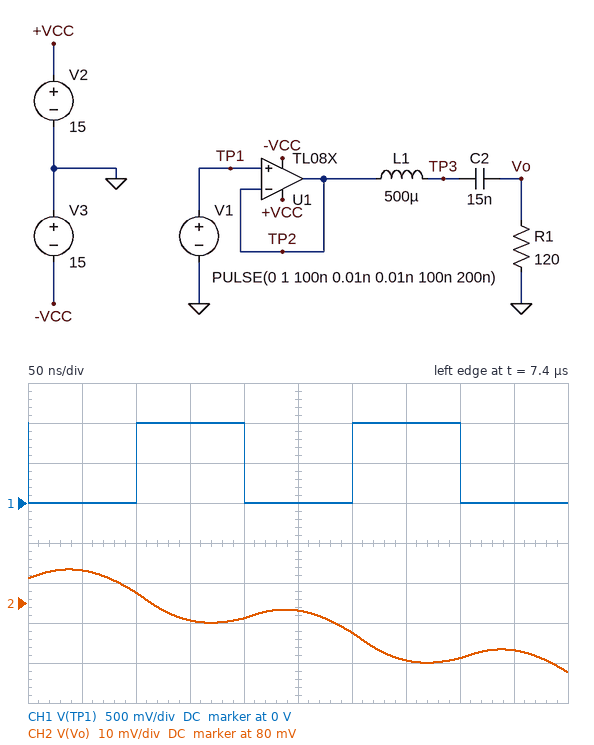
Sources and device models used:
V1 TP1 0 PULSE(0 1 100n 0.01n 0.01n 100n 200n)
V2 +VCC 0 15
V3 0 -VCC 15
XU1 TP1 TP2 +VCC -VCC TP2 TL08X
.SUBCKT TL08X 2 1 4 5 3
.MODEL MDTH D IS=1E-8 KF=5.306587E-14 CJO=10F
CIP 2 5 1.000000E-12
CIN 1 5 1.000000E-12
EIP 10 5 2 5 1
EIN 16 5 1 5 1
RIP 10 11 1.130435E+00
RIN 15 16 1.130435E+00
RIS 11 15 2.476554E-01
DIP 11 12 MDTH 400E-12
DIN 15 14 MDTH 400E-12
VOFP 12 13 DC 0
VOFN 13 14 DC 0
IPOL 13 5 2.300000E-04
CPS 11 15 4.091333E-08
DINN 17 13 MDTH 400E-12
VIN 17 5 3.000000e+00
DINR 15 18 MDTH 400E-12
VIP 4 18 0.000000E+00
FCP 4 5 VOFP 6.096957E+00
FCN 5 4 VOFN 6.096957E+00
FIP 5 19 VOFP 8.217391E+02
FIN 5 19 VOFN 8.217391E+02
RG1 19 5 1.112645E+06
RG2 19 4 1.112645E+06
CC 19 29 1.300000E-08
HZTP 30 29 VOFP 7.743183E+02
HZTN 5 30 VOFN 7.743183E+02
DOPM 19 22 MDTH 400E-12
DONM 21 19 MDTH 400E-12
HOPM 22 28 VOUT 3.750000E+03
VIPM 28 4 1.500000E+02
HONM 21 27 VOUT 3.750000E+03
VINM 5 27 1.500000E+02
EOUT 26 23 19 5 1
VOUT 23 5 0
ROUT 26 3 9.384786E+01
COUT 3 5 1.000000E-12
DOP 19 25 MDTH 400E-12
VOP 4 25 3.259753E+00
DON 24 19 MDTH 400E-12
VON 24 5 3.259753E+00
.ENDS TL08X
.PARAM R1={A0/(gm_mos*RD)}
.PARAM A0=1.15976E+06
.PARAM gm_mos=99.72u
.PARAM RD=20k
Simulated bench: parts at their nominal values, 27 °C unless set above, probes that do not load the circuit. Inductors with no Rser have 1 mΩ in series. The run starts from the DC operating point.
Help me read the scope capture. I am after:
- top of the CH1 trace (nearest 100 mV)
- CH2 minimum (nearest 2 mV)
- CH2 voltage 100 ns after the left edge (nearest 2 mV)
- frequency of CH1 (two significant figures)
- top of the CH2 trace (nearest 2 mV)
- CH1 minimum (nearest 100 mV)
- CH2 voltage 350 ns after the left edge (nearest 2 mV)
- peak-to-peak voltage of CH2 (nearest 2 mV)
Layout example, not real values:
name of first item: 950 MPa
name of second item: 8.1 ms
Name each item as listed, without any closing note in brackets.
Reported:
top of the CH1 trace: 1.0 V
CH2 minimum: 62 mV
CH2 voltage 100 ns after the left edge: 82 mV
frequency of CH1: 5.0 MHz
top of the CH2 trace: 88 mV
CH1 minimum: 0 V
CH2 voltage 350 ns after the left edge: 66 mV
peak-to-peak voltage of CH2: 26 mV
